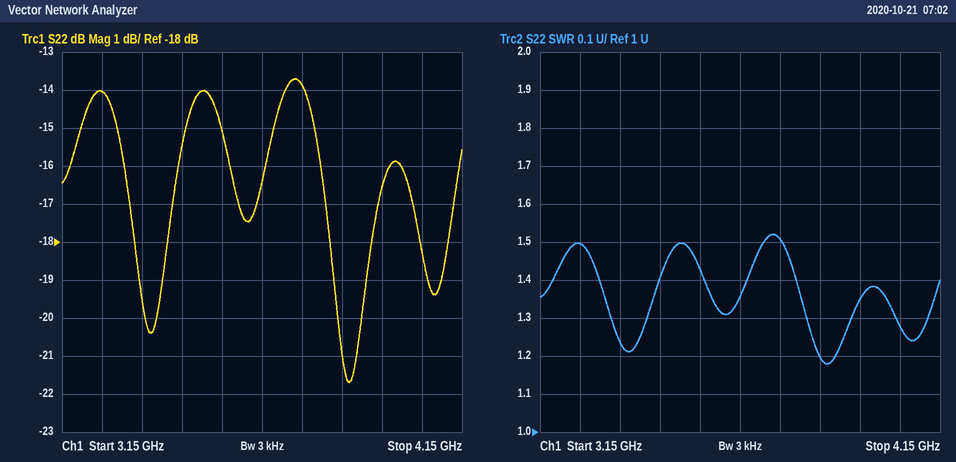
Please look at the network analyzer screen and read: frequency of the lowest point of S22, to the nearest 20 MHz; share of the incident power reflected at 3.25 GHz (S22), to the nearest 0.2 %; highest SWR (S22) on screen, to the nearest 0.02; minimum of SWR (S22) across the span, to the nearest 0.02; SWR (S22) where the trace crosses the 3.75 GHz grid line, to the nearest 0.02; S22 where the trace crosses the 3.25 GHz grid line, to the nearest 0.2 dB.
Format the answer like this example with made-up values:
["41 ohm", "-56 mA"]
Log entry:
["3.86 GHz", "4.0 %", "1.52", "1.18", "1.50", "-14.0 dB"]
